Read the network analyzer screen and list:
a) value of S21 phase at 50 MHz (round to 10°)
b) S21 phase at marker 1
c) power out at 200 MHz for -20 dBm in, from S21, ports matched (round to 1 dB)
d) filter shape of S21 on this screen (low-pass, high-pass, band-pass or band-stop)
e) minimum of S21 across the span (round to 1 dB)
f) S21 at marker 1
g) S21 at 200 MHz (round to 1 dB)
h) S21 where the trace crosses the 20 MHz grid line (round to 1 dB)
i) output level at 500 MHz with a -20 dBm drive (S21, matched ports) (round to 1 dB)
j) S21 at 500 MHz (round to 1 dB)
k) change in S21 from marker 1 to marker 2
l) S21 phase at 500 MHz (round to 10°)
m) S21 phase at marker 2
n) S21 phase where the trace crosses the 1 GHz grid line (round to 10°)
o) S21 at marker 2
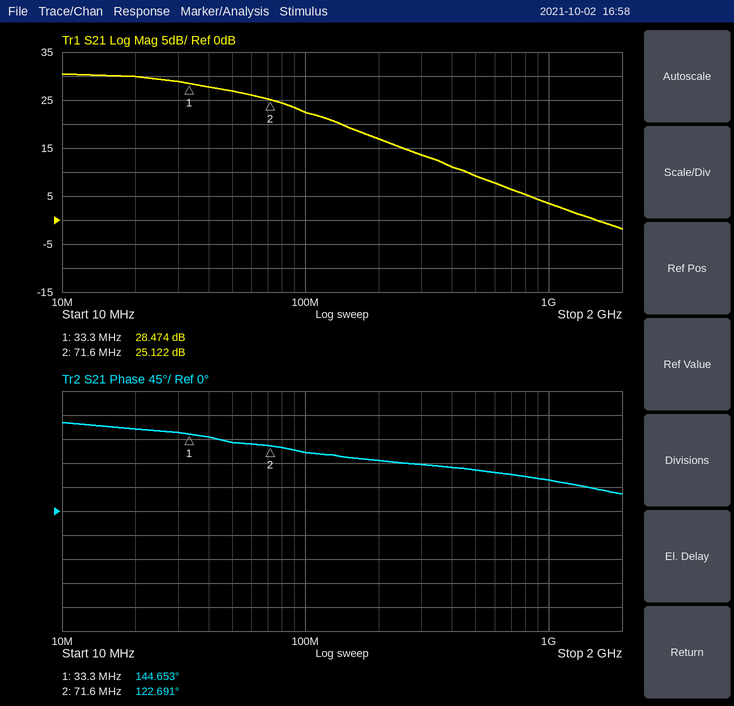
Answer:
130°
144.653°
-3 dBm
low-pass
-2 dB
28.474 dB
17 dB
30 dB
-11 dBm
9 dB
-3.352 dB
80°
122.691°
60°
25.122 dB
